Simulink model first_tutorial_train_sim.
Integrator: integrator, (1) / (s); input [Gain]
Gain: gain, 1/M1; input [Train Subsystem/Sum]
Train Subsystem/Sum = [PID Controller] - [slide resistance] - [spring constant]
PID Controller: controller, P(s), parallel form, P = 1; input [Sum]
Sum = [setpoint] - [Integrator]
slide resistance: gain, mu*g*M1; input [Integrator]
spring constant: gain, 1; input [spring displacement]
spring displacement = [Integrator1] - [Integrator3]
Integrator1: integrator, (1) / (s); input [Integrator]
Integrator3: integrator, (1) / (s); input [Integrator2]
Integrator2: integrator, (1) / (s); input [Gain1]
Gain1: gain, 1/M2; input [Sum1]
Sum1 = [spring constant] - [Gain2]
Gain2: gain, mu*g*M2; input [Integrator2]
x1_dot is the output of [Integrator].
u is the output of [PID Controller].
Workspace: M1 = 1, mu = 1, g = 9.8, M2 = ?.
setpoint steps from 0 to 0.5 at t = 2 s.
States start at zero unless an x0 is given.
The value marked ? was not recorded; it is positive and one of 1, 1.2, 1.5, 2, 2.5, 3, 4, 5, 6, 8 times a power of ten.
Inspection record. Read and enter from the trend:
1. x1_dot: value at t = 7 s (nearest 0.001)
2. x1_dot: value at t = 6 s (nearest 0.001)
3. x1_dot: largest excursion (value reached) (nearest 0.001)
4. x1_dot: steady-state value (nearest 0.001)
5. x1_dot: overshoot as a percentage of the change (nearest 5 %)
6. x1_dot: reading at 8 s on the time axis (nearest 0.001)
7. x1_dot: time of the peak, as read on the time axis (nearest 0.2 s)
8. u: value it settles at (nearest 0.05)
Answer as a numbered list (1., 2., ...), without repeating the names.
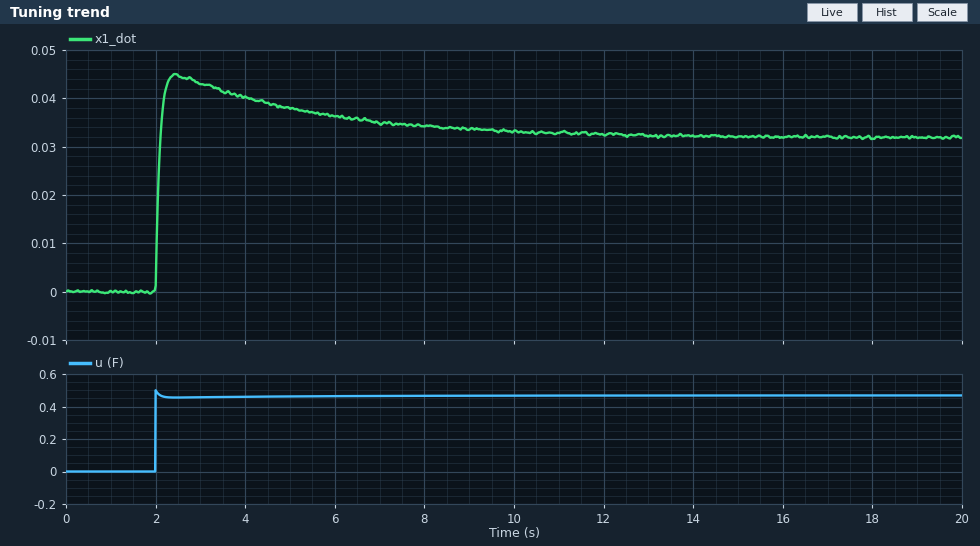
1. 0.035
2. 0.036
3. 0.045
4. 0.032
5. 40 %
6. 0.034
7. 2.4 s
8. 0.45
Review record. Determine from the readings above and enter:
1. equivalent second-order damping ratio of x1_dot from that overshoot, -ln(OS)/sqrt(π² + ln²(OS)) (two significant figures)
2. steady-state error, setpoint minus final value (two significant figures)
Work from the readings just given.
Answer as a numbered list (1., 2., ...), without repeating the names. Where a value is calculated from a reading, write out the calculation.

1. ln(0.4) = -0.916; 0.916 / sqrt(9.870 + 0.840) = 0.28
2. 0.5 - 0.032 = 0.47
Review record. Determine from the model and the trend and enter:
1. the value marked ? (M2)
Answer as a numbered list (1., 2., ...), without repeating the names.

1. 0.5
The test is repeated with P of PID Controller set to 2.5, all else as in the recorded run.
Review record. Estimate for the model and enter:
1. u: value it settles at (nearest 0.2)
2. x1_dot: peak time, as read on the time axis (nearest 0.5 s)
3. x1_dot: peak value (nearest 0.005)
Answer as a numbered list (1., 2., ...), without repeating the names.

1. 1.0
2. 2.5 s
3. 0.100
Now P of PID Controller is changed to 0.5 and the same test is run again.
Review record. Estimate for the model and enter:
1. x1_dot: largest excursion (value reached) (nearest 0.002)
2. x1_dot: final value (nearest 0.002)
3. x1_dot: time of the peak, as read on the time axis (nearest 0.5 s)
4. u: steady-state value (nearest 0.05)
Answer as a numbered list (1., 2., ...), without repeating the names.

1. 0.024
2. 0.016
3. 2.5 s
4. 0.25
